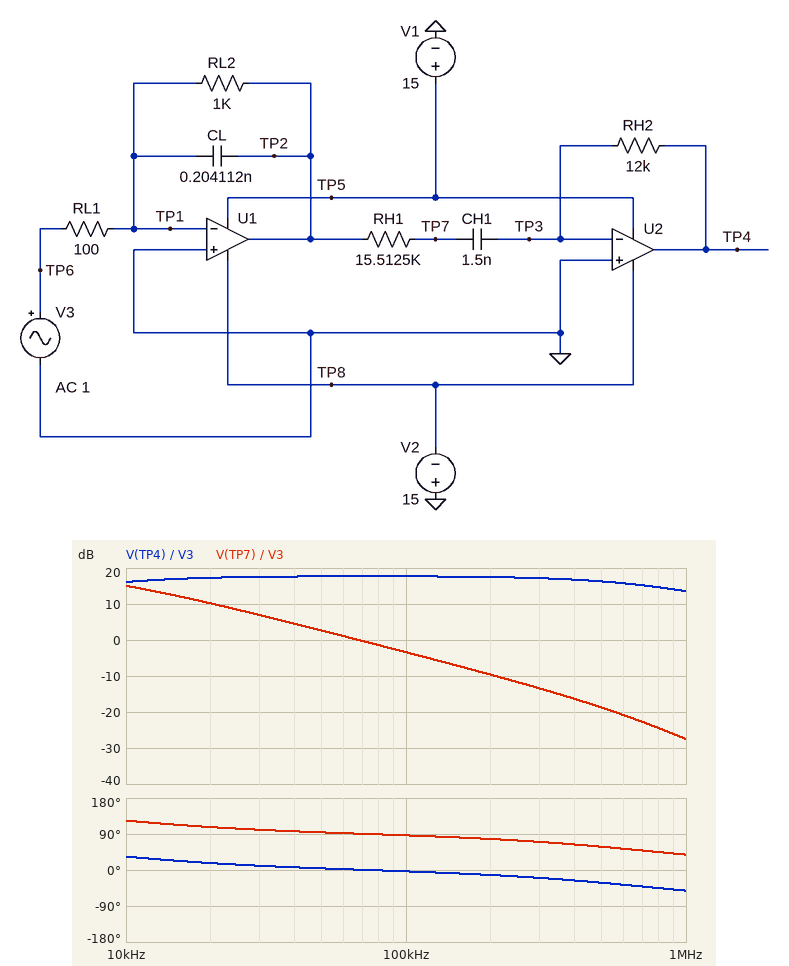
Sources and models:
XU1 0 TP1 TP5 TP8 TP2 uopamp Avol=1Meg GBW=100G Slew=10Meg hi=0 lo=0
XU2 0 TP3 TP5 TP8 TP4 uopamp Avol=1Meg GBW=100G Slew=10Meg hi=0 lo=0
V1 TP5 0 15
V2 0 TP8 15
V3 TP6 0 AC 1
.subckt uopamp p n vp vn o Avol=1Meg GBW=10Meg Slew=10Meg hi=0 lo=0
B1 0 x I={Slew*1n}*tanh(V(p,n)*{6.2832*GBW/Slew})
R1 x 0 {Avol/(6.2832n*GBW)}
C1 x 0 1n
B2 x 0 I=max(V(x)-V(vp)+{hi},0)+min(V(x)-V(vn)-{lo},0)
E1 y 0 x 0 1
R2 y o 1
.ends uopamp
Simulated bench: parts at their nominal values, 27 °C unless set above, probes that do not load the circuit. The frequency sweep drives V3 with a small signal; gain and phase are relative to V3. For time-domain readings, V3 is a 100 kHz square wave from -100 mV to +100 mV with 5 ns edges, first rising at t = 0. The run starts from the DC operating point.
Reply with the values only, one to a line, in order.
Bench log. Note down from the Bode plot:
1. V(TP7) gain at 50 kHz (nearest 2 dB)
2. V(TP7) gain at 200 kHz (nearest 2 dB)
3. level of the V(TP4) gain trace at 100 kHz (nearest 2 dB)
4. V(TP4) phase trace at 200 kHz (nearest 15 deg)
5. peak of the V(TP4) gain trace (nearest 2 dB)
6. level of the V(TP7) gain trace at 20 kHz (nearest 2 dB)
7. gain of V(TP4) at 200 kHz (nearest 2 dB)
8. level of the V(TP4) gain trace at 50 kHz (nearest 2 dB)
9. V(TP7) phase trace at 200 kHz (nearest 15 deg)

2 dB
-10 dB
18 dB
-15 deg
18 dB
10 dB
18 dB
18 dB
75 deg
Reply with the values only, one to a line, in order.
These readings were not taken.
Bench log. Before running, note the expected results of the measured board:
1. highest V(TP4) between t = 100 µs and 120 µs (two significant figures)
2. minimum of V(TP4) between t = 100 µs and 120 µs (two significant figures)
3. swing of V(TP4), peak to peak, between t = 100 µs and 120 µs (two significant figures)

830 mV
-810 mV
1.6 V
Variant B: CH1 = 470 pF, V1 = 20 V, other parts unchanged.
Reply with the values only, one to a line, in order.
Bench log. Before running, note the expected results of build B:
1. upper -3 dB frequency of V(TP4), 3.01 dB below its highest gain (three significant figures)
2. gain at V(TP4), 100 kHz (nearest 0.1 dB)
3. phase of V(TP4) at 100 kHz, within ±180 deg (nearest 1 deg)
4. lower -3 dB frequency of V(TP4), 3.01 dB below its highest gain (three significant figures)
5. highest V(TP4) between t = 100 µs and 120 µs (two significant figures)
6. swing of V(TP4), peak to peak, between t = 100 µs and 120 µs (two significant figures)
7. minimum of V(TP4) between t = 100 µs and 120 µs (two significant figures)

822 kHz
17.5 dB
5 deg
20.7 kHz
920 mV
1.8 V
-920 mV
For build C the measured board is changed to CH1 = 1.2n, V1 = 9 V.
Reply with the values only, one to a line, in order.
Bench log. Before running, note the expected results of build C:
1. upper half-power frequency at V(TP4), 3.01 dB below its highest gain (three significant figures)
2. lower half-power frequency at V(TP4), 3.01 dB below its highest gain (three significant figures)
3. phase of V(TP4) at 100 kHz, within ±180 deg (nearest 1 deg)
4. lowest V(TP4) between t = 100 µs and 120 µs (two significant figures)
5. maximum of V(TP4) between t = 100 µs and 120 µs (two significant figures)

797 kHz
8.37 kHz
-2 deg
-830 mV
830 mV
